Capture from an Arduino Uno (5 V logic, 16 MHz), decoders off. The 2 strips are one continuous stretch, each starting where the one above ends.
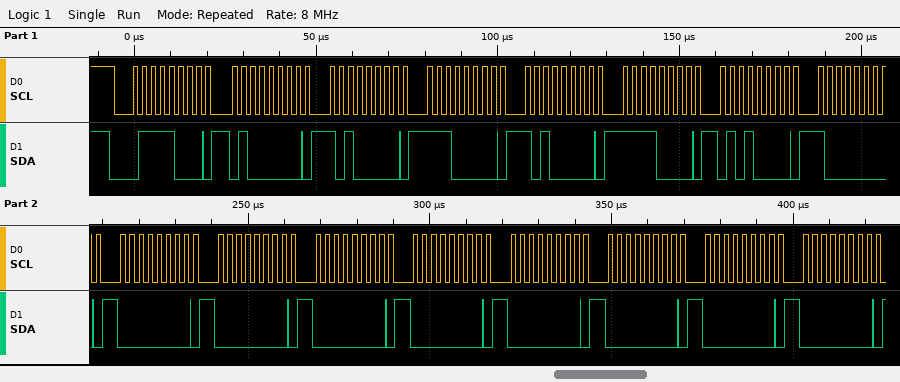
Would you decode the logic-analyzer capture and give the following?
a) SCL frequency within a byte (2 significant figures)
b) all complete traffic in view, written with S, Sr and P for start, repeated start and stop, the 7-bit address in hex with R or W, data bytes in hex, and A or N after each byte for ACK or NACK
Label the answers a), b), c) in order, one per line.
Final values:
a) 400 kHz
b) S 3CW A 40 A A0 A E0 A A0 A F0 A 50 A 80 A 00 A 00 A 00 A 00 A 00 A 00 A 00 A 00 A
